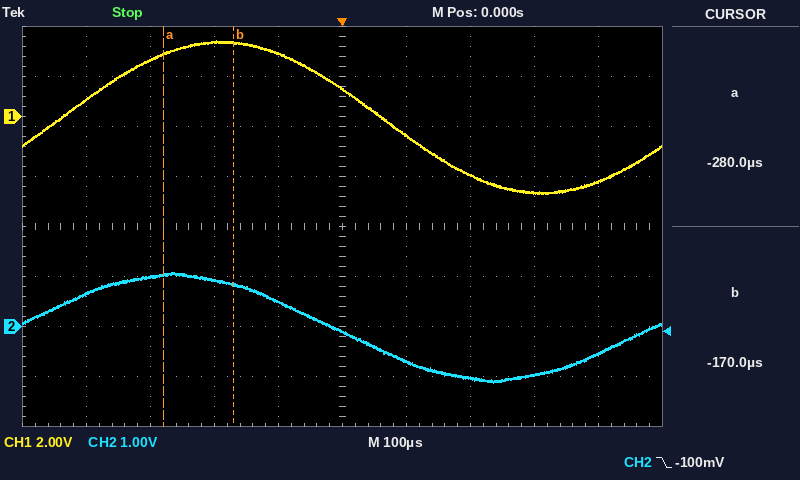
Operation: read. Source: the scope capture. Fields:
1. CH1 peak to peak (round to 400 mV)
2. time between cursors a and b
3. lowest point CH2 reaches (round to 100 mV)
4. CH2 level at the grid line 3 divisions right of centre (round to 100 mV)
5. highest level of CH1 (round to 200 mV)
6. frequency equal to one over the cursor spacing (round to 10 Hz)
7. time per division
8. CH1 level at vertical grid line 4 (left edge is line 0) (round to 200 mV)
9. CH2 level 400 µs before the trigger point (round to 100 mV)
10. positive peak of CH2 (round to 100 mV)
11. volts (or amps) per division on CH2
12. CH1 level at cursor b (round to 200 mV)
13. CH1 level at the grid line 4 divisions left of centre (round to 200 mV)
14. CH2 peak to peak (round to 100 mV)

6.0 V
110 µs
-1.1 V
-1.0 V
3.0 V
9.09 kHz
100 µs
2.6 V
700 mV
1.1 V
1 V
3.0 V
600 mV
2.2 V
